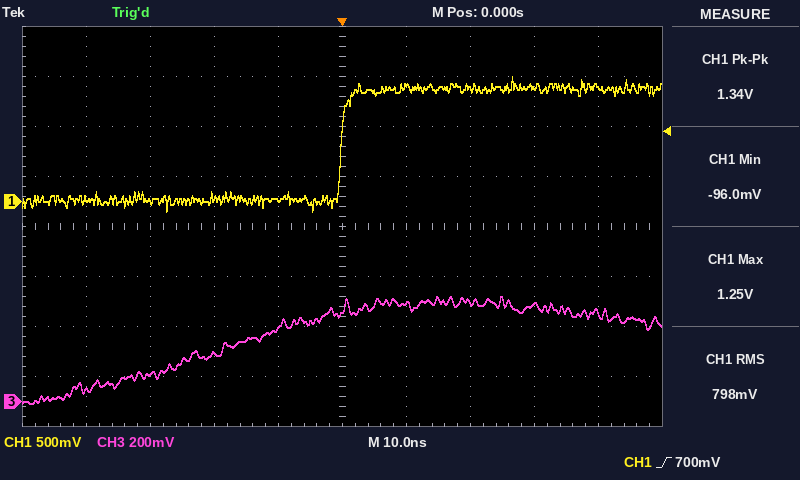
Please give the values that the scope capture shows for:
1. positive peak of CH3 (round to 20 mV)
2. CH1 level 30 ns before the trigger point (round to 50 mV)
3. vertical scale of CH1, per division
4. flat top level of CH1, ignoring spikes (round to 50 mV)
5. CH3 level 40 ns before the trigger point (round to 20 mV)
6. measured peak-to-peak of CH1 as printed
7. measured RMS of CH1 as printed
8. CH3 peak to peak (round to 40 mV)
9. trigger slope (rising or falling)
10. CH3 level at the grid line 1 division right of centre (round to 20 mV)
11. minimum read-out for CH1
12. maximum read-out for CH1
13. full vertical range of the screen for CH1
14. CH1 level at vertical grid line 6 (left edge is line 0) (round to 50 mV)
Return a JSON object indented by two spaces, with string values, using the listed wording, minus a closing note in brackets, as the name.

{
  "positive peak of CH3": "420 mV",
  "CH1 level 30 ns before the trigger point": "0 mV",
  "vertical scale of CH1, per division": "500 mV",
  "flat top level of CH1, ignoring spikes": "1.15 V",
  "CH3 level 40 ns before the trigger point": "40 mV",
  "measured peak-to-peak of CH1 as printed": "1.34 V",
  "measured RMS of CH1 as printed": "798 mV",
  "CH3 peak to peak": "440 mV",
  "trigger slope": "rising",
  "CH3 level at the grid line 1 division right of centre": "400 mV",
  "minimum read-out for CH1": "-96.0 mV",
  "maximum read-out for CH1": "1.25 V",
  "full vertical range of the screen for CH1": "4 V",
  "CH1 level at vertical grid line 6 (left edge is line 0)": "1.15 V"
}
